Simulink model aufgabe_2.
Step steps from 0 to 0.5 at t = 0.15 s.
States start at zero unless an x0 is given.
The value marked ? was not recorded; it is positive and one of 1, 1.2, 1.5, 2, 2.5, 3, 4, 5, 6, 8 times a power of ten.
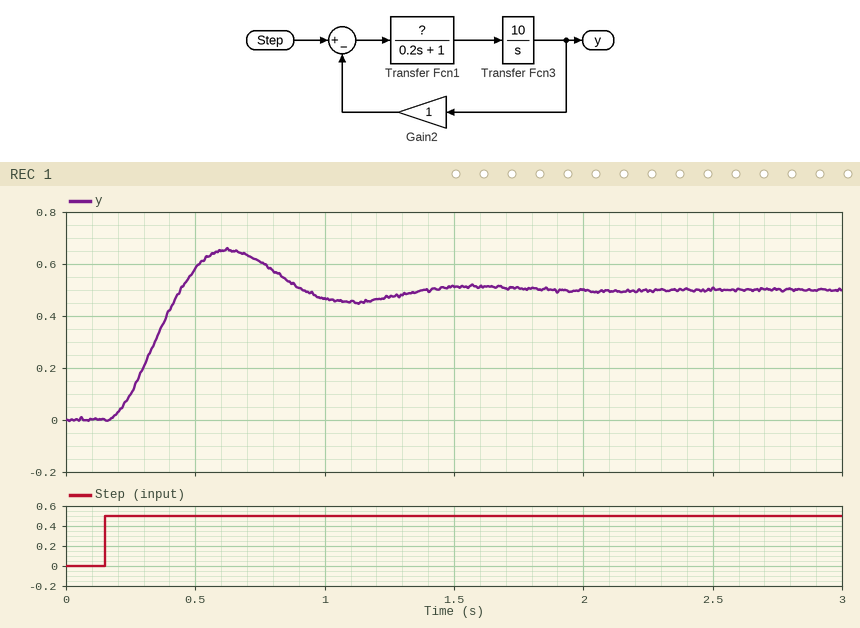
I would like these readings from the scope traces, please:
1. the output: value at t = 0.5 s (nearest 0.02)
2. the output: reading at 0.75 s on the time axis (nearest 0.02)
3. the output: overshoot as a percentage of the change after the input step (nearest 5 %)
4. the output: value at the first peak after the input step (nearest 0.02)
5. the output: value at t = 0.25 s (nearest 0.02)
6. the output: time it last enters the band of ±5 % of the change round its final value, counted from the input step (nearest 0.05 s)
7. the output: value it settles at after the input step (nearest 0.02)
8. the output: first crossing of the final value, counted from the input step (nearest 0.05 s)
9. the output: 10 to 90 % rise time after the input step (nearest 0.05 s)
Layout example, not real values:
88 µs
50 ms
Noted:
0.58
0.60
30 %
0.66
0.10
1.10 s
0.50
0.30 s
0.20 s
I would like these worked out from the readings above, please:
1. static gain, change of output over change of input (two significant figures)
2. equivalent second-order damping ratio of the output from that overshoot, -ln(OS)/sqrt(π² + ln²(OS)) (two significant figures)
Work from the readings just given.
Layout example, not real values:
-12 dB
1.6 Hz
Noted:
1.0
0.36
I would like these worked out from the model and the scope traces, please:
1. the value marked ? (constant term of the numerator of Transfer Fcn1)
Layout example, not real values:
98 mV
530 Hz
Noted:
1
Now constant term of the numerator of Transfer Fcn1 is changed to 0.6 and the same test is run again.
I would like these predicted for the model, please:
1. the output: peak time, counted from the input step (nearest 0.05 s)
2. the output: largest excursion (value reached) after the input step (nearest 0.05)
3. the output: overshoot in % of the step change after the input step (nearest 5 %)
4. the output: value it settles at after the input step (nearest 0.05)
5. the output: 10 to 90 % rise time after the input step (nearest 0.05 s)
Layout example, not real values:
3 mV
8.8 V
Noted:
0.65 s
0.60
20 %
0.50
0.30 s
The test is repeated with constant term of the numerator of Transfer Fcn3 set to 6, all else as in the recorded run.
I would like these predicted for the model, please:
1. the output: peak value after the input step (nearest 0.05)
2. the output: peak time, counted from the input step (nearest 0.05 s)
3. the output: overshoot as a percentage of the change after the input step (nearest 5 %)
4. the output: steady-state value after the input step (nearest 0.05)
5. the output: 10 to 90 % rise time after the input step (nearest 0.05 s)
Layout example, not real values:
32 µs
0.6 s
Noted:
0.60
0.65 s
20 %
0.50
0.30 s
